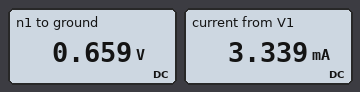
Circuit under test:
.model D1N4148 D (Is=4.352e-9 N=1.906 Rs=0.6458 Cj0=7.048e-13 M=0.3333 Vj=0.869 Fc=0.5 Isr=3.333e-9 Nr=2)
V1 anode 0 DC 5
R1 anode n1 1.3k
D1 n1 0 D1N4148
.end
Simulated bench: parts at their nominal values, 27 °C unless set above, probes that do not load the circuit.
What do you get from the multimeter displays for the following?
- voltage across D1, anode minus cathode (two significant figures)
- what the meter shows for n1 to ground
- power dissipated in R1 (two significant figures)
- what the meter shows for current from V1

660 mV
0.659 V
14 mW
3.339 mA
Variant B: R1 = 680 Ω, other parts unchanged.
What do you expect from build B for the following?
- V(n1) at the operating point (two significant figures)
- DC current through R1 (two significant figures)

690 mV
6.3 mA
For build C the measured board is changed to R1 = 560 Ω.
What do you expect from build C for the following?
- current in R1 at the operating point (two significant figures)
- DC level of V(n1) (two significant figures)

7.7 mA
700 mV
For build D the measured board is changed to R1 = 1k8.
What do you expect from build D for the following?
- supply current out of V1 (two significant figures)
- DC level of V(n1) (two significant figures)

2.4 mA
640 mV
